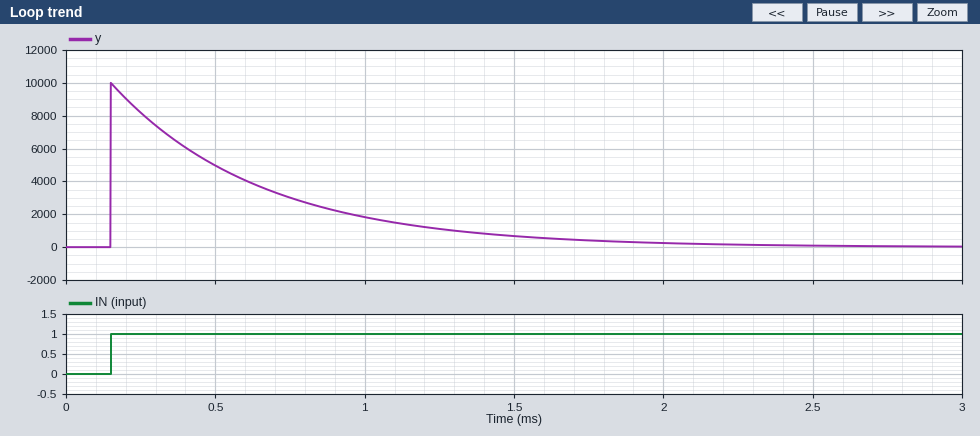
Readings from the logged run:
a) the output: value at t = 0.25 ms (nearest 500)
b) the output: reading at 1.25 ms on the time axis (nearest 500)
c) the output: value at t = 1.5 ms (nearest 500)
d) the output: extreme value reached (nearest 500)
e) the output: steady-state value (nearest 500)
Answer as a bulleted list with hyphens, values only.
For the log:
- 8000
- 1000
- 500
- 10000
- 0
